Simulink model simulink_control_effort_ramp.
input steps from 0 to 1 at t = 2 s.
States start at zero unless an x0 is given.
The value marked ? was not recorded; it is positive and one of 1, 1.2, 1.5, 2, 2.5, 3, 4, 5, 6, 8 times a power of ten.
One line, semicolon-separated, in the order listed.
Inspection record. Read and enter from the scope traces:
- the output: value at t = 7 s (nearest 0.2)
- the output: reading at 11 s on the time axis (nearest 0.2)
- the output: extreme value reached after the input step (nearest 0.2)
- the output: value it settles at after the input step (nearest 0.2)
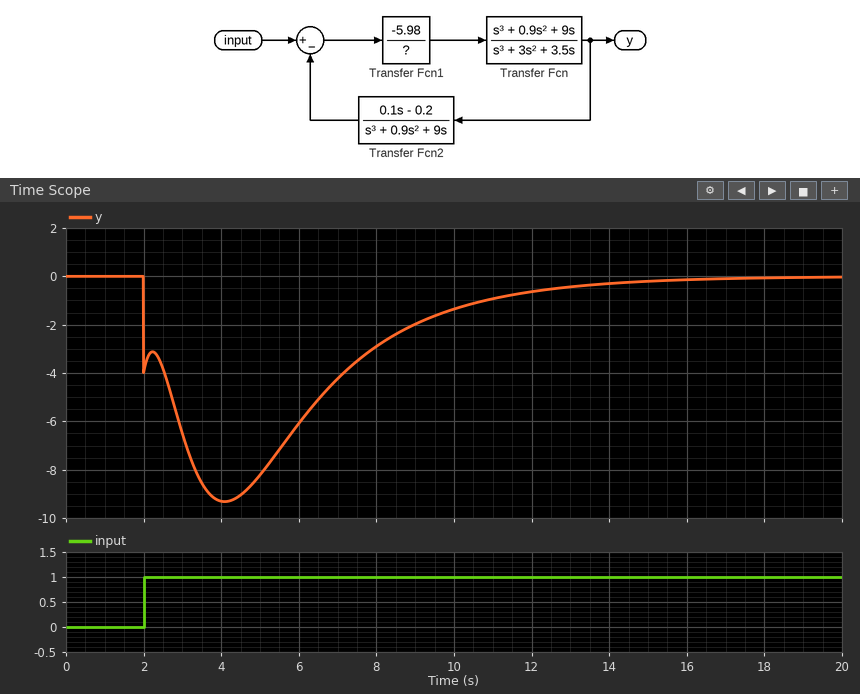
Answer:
-4.2; -1.0; -9.4; 0.0
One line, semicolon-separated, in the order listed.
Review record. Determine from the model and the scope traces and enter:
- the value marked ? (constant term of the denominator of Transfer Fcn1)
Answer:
1.5
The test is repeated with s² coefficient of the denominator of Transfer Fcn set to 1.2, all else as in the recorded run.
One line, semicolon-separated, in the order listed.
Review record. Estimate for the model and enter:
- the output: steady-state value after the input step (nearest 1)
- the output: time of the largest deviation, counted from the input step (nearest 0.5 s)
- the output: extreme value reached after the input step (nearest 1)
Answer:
0; 1.5 s; -12
